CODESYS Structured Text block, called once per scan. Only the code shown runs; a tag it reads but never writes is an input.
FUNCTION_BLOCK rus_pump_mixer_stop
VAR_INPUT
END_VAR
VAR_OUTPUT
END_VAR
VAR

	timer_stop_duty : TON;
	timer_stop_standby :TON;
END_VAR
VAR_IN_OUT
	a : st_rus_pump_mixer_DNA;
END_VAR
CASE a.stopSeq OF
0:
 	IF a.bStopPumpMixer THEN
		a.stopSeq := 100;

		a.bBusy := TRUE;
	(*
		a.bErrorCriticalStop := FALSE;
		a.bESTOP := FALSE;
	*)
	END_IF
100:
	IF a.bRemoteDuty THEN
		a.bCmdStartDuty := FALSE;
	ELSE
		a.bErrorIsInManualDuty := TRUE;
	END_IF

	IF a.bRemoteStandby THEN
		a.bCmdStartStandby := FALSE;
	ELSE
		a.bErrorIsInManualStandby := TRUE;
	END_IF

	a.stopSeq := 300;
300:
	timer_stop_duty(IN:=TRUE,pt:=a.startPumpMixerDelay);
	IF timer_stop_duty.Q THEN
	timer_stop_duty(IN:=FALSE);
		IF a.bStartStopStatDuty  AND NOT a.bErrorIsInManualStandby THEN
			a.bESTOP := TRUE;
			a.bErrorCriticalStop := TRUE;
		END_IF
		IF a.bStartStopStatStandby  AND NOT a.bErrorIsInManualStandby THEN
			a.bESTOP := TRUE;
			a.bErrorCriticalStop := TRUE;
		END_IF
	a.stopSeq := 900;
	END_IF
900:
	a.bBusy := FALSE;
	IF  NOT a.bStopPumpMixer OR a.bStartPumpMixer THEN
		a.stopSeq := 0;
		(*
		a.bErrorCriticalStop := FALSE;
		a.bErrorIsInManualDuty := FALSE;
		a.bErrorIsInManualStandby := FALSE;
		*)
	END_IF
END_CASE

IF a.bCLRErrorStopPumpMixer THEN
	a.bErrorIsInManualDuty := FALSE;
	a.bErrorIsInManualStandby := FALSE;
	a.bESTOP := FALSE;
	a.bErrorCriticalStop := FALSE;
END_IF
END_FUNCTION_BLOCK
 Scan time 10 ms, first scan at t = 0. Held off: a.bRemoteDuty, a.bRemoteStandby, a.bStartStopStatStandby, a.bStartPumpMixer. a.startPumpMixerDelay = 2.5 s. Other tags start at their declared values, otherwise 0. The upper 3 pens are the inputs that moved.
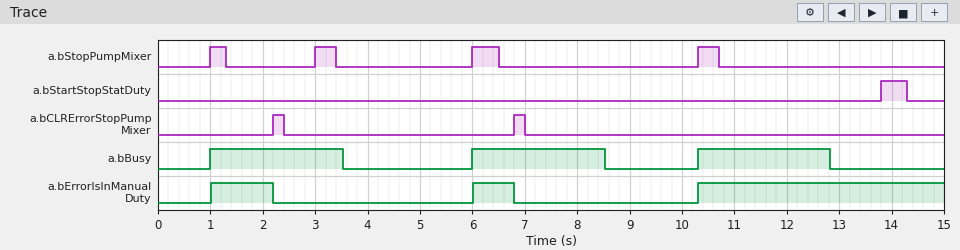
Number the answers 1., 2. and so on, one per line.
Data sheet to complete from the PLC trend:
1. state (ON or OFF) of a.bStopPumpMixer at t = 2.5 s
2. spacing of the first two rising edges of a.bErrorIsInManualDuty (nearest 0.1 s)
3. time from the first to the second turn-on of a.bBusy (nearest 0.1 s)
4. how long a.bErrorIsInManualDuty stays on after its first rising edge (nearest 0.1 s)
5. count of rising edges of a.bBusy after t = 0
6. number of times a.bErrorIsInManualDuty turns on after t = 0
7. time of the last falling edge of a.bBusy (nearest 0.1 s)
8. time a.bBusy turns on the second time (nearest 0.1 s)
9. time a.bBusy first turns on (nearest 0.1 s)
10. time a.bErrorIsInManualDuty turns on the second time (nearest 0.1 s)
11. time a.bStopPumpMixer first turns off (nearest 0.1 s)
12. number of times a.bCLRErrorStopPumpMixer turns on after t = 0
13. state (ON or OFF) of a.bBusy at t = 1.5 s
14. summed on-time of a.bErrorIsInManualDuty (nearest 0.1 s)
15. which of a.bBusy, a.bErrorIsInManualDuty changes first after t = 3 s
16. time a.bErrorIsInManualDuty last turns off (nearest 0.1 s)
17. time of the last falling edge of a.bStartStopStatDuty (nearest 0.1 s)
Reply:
1. OFF
2. 5.0 s
3. 5.0 s
4. 1.2 s
5. 3
6. 3
7. 12.8 s
8. 6.0 s
9. 1.0 s
10. 6.0 s
11. 1.3 s
12. 2
13. ON
14. 6.7 s
15. a.bBusy
16. 6.8 s
17. 14.3 s
